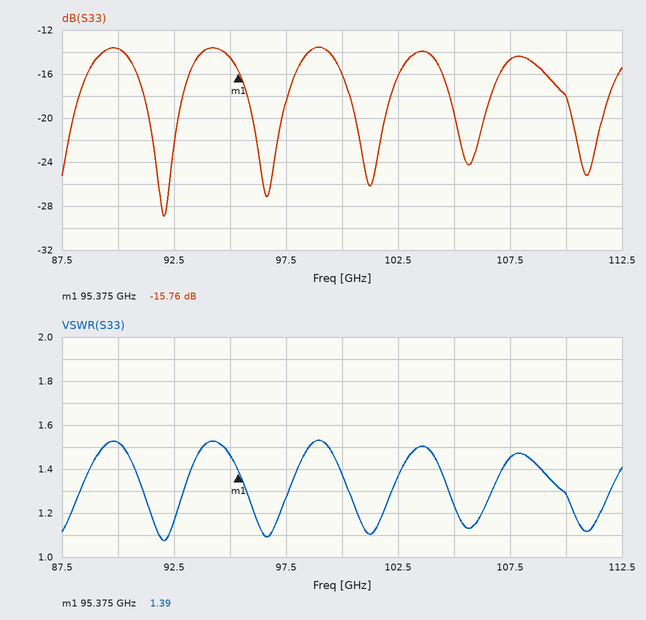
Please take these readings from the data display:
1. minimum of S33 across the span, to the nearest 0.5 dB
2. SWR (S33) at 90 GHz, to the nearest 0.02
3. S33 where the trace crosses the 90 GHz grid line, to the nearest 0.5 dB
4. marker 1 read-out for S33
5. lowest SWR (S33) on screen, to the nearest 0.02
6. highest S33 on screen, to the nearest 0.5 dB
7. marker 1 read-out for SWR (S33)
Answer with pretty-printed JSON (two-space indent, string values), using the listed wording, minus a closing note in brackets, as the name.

{
  "minimum of S33 across the span, to the nearest 0.5 dB": "-29.0 dB",
  "SWR (S33) at 90 GHz, to the nearest 0.02": "1.52",
  "S33 where the trace crosses the 90 GHz grid line, to the nearest 0.5 dB": "-13.5 dB",
  "marker 1 read-out for S33": "-15.76 dB",
  "lowest SWR (S33) on screen, to the nearest 0.02": "1.08",
  "highest S33 on screen, to the nearest 0.5 dB": "-13.5 dB",
  "marker 1 read-out for SWR": "1.39"
}
